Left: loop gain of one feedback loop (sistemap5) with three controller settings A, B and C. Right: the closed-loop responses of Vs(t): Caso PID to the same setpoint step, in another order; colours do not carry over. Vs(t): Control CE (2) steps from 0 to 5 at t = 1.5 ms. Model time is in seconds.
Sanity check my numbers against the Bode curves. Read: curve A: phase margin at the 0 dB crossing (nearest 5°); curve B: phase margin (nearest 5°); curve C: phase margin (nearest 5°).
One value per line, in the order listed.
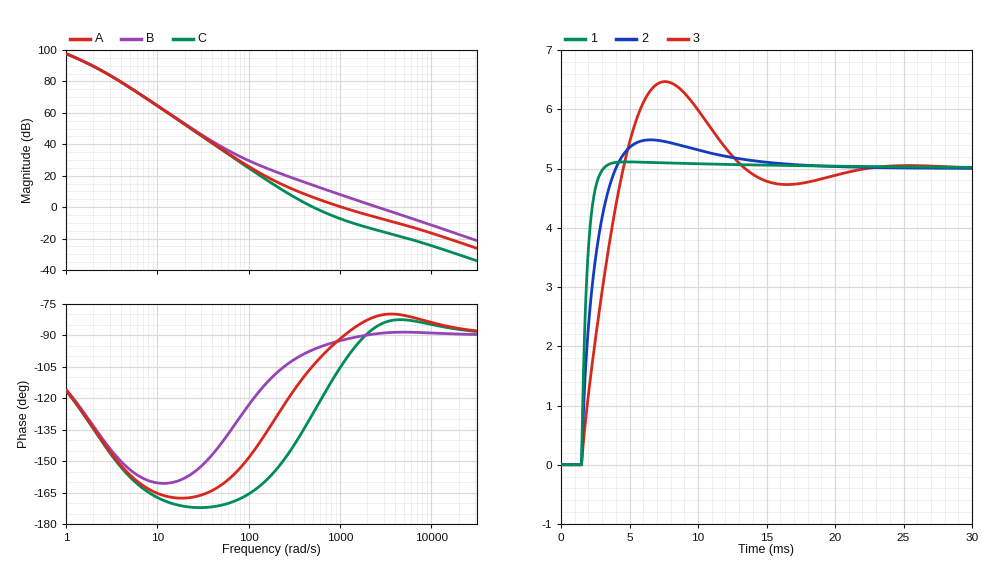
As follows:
90°
90°
55°
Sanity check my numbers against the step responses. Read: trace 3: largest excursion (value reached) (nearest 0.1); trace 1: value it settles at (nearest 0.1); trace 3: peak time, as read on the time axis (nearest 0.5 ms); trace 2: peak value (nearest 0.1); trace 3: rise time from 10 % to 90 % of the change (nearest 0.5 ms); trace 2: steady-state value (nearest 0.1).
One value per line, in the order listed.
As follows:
6.5
5.0
7.5 ms
5.5
2.5 ms
5.0
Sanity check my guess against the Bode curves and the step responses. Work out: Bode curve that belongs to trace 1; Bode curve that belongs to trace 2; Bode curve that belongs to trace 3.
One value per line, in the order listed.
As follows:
B
A
C
